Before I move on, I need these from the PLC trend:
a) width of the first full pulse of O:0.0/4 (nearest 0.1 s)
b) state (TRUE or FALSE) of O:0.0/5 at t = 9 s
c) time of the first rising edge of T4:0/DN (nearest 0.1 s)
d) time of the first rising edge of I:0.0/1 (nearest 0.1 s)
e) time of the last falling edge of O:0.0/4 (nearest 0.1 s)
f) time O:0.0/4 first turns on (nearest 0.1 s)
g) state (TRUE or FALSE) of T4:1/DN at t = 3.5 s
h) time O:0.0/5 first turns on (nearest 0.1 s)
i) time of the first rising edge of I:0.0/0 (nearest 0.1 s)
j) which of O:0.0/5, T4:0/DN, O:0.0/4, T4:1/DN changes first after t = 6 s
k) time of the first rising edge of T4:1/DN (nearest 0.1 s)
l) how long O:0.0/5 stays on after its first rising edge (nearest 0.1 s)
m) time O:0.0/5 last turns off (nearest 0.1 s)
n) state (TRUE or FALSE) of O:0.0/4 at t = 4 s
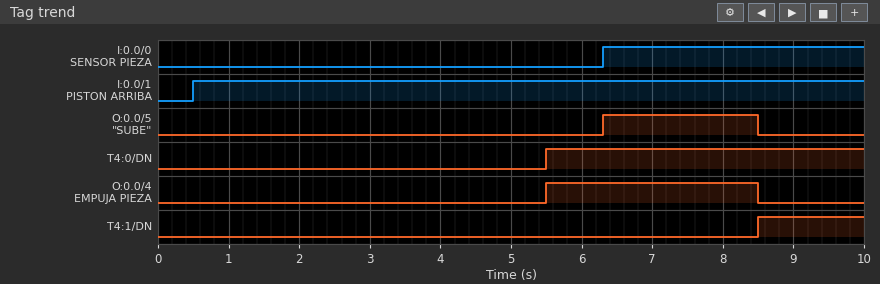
3.0 s
FALSE
5.5 s
0.5 s
8.5 s
5.5 s
FALSE
6.3 s
6.3 s
O:0.0/5
8.5 s
2.2 s
8.5 s
FALSE
